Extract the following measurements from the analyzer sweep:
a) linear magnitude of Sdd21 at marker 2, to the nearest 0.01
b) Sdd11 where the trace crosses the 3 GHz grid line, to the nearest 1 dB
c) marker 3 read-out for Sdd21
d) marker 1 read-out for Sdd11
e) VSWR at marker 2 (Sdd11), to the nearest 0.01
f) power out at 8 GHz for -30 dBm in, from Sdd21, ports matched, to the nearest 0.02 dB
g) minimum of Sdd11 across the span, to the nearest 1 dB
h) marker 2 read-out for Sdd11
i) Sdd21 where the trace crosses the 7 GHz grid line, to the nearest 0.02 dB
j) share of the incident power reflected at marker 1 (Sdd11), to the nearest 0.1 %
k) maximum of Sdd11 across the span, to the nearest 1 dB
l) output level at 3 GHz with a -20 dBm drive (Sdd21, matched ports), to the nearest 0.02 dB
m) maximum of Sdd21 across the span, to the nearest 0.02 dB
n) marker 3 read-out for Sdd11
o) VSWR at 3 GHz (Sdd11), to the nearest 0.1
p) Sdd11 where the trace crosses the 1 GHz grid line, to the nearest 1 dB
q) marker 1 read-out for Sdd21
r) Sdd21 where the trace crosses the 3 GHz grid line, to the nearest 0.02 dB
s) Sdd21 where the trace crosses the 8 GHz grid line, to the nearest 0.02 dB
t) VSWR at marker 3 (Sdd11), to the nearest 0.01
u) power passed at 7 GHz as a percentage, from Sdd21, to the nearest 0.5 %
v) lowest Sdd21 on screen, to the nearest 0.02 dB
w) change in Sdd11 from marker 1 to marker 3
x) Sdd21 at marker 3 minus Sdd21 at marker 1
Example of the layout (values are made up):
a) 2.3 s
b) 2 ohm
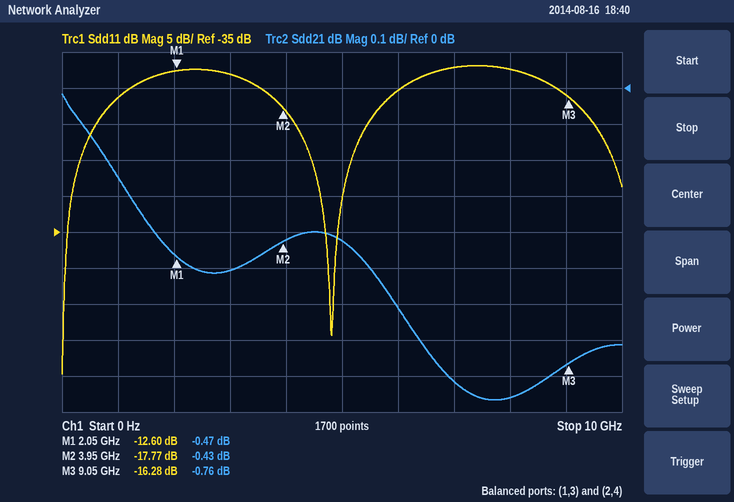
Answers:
a) 0.95
b) -13 dB
c) -0.76 dB
d) -12.60 dB
e) 1.30
f) -30.86 dBm
g) -55 dB
h) -17.77 dB
i) -0.82 dB
j) 5.5 %
k) -12 dB
l) -20.50 dBm
m) -0.02 dB
n) -16.28 dB
o) 1.6
p) -16 dB
q) -0.47 dB
r) -0.50 dB
s) -0.86 dB
t) 1.36
u) 83.0 %
v) -0.86 dB
w) -3.68 dB
x) -0.29 dB
